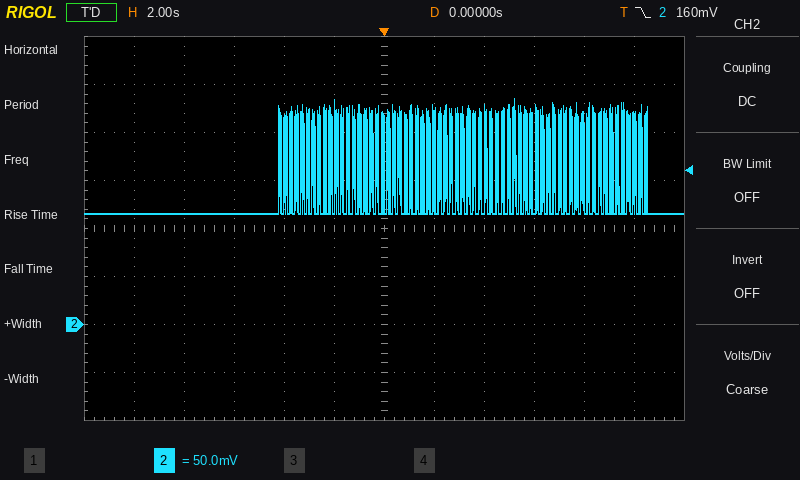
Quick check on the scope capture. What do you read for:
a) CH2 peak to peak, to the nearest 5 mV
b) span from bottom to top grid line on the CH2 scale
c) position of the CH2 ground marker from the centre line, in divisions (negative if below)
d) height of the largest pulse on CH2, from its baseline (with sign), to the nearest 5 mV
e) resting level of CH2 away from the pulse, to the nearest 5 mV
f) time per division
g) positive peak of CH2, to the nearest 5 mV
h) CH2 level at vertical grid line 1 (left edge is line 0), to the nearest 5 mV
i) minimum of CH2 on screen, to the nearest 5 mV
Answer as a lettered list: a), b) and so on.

a) 120 mV
b) 400 mV
c) -2.0 div
d) +120 mV
e) 115 mV
f) 2 s
g) 235 mV
h) 115 mV
i) 115 mV
